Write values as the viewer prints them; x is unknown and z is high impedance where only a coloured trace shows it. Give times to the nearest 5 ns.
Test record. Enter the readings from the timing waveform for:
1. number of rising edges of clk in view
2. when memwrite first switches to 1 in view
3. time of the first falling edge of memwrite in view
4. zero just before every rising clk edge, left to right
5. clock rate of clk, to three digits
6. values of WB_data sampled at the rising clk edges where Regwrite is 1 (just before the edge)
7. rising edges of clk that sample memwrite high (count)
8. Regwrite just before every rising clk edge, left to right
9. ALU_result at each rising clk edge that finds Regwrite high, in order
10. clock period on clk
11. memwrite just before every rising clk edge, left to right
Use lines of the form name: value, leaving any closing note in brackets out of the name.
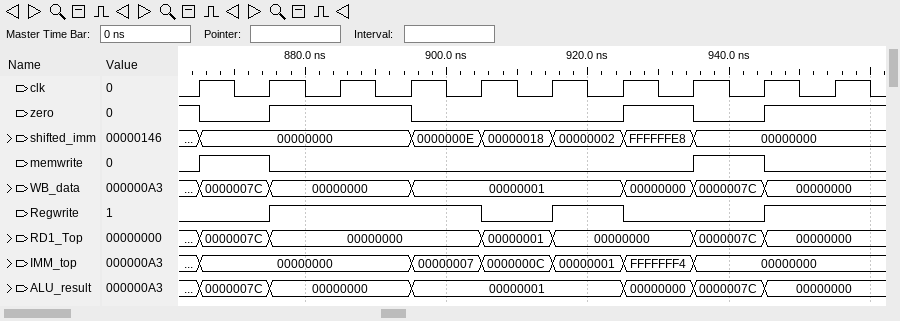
number of rising edges of clk in view: 10
when memwrite first switches to 1 in view: 865 ns
time of the first falling edge of memwrite in view: 875 ns
zero just before every rising clk edge, left to right: 1 0 1 1 0 0 0 1 0 1
clock rate of clk, to three digits: 100 MHz
values of WB_data sampled at the rising clk edges where Regwrite is 1: 00000000, 00000000, 00000001, 00000001, 00000000
rising edges of clk that sample memwrite high: 2
Regwrite just before every rising clk edge, left to right: 0 0 1 1 1 0 1 0 0 1
ALU_result at each rising clk edge that finds Regwrite high, in order: 00000000, 00000000, 00000001, 00000001, 00000000
clock period on clk: 10 ns
memwrite just before every rising clk edge, left to right: 0 1 0 0 0 0 0 0 1 0
